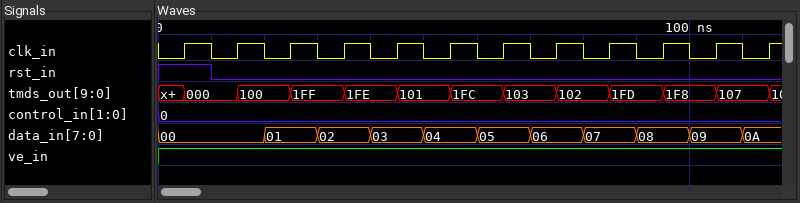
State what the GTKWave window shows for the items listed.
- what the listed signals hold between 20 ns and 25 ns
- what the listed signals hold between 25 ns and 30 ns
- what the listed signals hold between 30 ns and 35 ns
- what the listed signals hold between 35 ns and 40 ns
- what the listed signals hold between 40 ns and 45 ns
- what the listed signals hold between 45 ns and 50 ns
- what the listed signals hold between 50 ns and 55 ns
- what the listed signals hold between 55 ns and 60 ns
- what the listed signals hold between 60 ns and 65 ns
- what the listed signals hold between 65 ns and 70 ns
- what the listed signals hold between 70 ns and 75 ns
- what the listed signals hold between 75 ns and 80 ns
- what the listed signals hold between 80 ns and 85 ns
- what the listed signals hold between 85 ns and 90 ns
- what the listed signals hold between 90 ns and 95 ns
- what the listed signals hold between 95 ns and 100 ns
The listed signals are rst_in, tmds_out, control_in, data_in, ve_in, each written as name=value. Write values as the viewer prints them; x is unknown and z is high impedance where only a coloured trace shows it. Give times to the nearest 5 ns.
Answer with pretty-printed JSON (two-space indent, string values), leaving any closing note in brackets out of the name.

{
  "what the listed signals hold between 20 ns and 25 ns": "rst_in=0, tmds_out=100, control_in=0, data_in=01, ve_in=1",
  "what the listed signals hold between 25 ns and 30 ns": "rst_in=0, tmds_out=1FF, control_in=0, data_in=01, ve_in=1",
  "what the listed signals hold between 30 ns and 35 ns": "rst_in=0, tmds_out=1FF, control_in=0, data_in=02, ve_in=1",
  "what the listed signals hold between 35 ns and 40 ns": "rst_in=0, tmds_out=1FE, control_in=0, data_in=02, ve_in=1",
  "what the listed signals hold between 40 ns and 45 ns": "rst_in=0, tmds_out=1FE, control_in=0, data_in=03, ve_in=1",
  "what the listed signals hold between 45 ns and 50 ns": "rst_in=0, tmds_out=101, control_in=0, data_in=03, ve_in=1",
  "what the listed signals hold between 50 ns and 55 ns": "rst_in=0, tmds_out=101, control_in=0, data_in=04, ve_in=1",
  "what the listed signals hold between 55 ns and 60 ns": "rst_in=0, tmds_out=1FC, control_in=0, data_in=04, ve_in=1",
  "what the listed signals hold between 60 ns and 65 ns": "rst_in=0, tmds_out=1FC, control_in=0, data_in=05, ve_in=1",
  "what the listed signals hold between 65 ns and 70 ns": "rst_in=0, tmds_out=103, control_in=0, data_in=05, ve_in=1",
  "what the listed signals hold between 70 ns and 75 ns": "rst_in=0, tmds_out=103, control_in=0, data_in=06, ve_in=1",
  "what the listed signals hold between 75 ns and 80 ns": "rst_in=0, tmds_out=102, control_in=0, data_in=06, ve_in=1",
  "what the listed signals hold between 80 ns and 85 ns": "rst_in=0, tmds_out=102, control_in=0, data_in=07, ve_in=1",
  "what the listed signals hold between 85 ns and 90 ns": "rst_in=0, tmds_out=1FD, control_in=0, data_in=07, ve_in=1",
  "what the listed signals hold between 90 ns and 95 ns": "rst_in=0, tmds_out=1FD, control_in=0, data_in=08, ve_in=1",
  "what the listed signals hold between 95 ns and 100 ns": "rst_in=0, tmds_out=1F8, control_in=0, data_in=08, ve_in=1"
}
